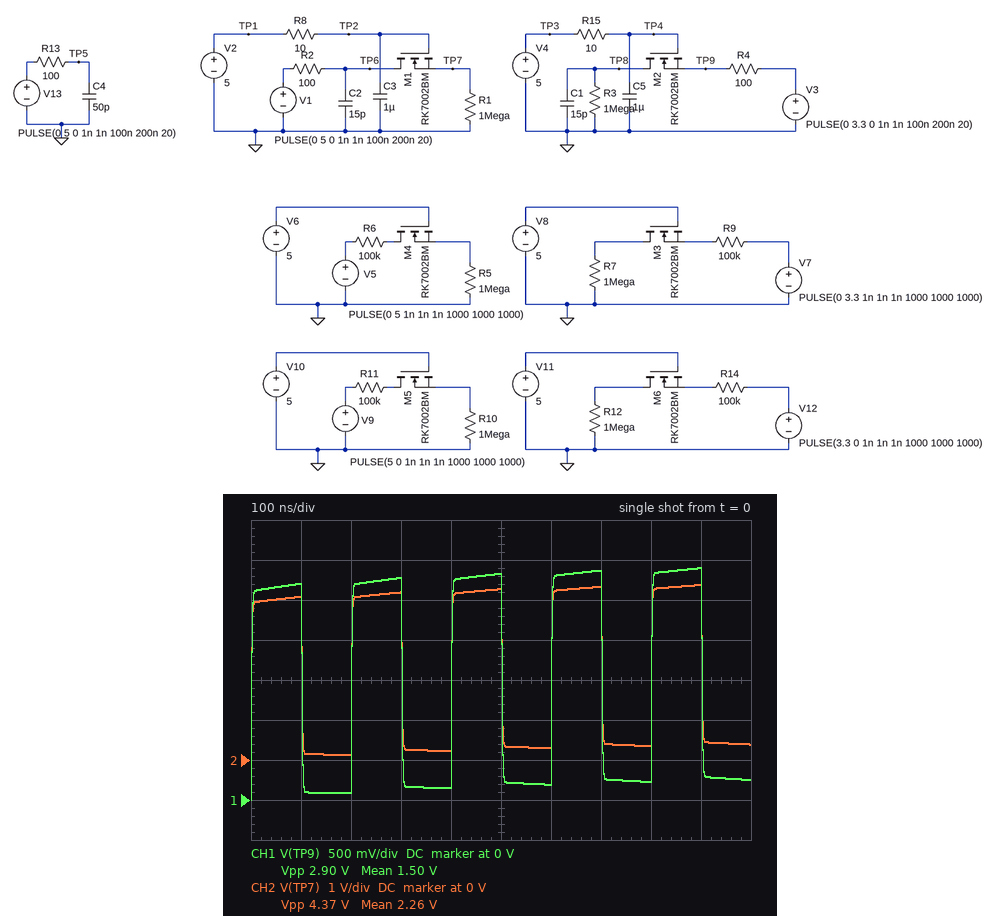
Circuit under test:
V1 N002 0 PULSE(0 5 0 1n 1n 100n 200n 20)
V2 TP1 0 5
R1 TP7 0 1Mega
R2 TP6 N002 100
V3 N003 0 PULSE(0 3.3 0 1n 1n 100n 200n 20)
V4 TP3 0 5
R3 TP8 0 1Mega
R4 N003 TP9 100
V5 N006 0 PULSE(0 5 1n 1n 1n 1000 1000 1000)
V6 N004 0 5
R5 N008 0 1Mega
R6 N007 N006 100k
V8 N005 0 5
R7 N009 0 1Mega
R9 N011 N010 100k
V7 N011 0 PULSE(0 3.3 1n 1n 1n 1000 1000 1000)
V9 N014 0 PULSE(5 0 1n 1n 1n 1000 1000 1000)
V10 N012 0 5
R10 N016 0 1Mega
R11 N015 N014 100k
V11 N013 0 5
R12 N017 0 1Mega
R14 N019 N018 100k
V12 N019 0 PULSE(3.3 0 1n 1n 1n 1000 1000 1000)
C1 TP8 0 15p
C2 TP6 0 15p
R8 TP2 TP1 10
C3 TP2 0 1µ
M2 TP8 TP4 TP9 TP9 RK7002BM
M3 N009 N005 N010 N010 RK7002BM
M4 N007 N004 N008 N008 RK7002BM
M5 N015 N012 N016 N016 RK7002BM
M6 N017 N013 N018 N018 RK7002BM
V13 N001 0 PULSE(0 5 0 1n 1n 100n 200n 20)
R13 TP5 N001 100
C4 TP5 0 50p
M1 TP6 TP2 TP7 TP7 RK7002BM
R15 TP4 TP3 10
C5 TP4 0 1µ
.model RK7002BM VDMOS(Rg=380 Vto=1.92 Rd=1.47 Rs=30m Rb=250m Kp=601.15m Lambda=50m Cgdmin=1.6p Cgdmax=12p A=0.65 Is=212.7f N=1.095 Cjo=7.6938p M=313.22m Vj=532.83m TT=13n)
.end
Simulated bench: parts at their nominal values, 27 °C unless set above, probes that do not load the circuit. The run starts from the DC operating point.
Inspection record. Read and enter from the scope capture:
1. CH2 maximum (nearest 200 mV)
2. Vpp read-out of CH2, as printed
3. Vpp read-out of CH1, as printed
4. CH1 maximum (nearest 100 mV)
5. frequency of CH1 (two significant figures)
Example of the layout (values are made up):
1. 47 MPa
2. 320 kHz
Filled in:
1. 4.4 V
2. 4.37 V
3. 2.90 V
4. 2.9 V
5. 5.0 MHz
